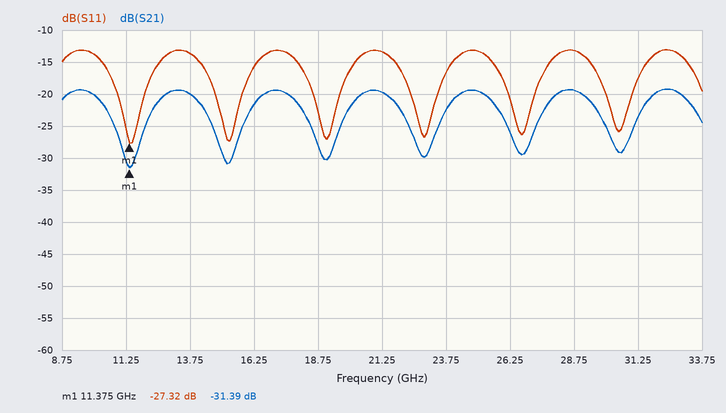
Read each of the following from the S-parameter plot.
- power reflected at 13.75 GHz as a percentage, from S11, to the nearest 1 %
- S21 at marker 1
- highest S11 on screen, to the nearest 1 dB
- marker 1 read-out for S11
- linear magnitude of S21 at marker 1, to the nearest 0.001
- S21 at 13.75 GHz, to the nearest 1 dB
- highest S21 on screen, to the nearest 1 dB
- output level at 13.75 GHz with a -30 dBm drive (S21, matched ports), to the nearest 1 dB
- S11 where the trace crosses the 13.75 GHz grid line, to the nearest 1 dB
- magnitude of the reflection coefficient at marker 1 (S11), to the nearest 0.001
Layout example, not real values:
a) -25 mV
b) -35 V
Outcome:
a) 4 %
b) -31.39 dB
c) -13 dB
d) -27.32 dB
e) 0.027
f) -20 dB
g) -19 dB
h) -50 dBm
i) -14 dB
j) 0.043
